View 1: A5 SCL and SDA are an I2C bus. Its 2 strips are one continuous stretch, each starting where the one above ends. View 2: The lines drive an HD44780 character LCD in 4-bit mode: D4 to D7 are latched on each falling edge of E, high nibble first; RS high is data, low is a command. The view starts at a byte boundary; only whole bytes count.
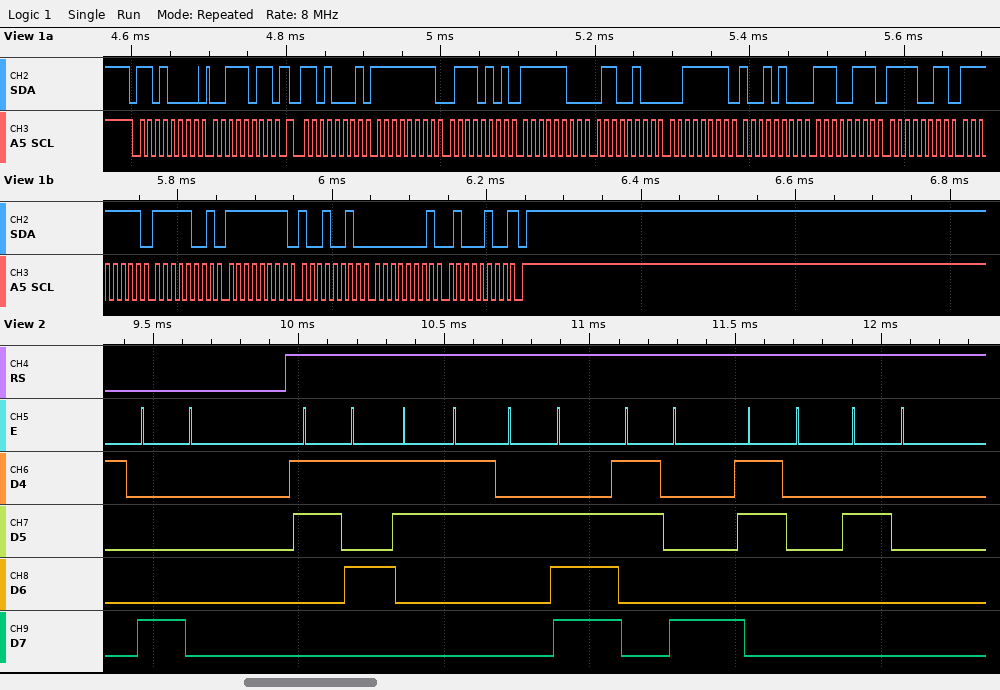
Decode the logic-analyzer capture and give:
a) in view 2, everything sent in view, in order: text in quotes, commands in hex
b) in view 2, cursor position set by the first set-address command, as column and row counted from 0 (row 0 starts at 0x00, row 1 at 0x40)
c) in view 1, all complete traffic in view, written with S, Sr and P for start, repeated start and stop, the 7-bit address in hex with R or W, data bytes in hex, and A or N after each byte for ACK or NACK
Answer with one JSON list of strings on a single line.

["0x80 \"53.80 \"", "column 0, row 0", "S 68W A 3B A Sr 68R A FF A 75 A FC A 64 A 3F A 94 A E7 A F3 A FF A F9 A FF A 92 A 01 A 44 N P"]
